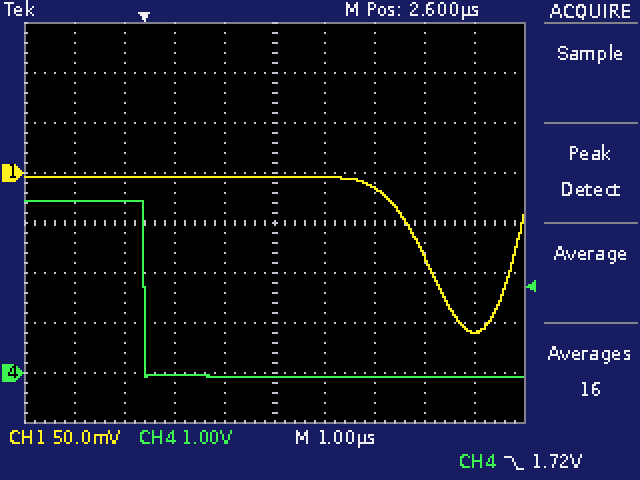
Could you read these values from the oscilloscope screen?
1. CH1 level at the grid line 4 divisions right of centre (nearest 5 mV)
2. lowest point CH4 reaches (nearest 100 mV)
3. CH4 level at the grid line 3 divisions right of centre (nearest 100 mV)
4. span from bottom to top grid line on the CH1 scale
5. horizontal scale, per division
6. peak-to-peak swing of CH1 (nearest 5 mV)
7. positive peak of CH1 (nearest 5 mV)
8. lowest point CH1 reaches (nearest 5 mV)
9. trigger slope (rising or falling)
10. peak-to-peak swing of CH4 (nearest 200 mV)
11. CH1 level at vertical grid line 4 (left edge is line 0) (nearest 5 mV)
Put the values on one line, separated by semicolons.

-160 mV; -100 mV; -100 mV; 400 mV; 1 µs; 155 mV; -5 mV; -160 mV; falling; 3.6 V; -5 mV
